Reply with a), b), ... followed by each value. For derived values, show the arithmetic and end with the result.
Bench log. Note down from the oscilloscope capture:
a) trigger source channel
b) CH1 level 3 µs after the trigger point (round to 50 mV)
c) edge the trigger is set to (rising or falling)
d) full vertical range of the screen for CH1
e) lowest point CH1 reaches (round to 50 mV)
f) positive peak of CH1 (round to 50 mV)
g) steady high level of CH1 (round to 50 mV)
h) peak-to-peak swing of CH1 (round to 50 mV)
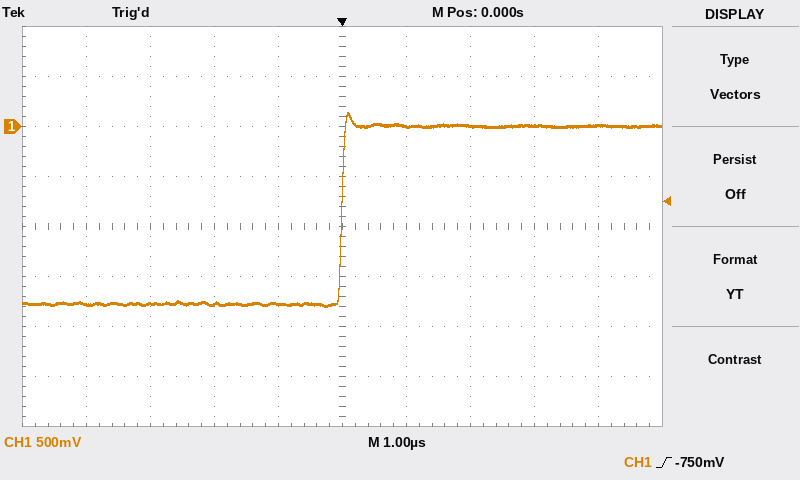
a) CH1
b) 0 mV
c) rising
d) 4 V
e) -1.80 V
f) 150 mV
g) 0 mV
h) 150 mV − (-1.80 V) = 1.95 V
